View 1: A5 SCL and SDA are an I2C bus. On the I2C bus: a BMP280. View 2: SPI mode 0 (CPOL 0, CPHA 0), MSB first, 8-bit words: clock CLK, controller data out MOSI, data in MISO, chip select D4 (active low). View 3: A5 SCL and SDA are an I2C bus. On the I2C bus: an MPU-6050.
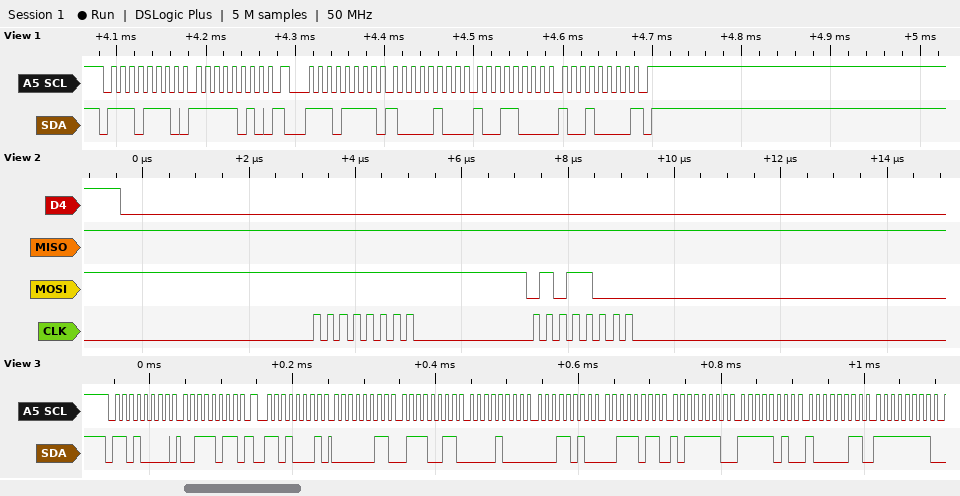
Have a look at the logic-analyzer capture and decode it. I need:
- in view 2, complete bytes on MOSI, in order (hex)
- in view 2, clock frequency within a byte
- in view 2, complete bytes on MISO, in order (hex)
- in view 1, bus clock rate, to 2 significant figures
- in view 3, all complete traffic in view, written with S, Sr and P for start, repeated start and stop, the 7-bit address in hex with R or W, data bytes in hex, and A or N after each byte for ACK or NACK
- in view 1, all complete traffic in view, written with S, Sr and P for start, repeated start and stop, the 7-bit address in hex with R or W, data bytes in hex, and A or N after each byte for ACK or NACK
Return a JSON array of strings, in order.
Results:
["0xFF 0x58", "4 MHz", "0xFF 0xFF", "100 kHz", "S 68W A 3B A Sr 68R A 03 A 73 A 08 A 1A A 3B A BE A FA A 83 A FF A", "S 77W A FA A Sr 77R A 84 A 98 A 90 N P"]
